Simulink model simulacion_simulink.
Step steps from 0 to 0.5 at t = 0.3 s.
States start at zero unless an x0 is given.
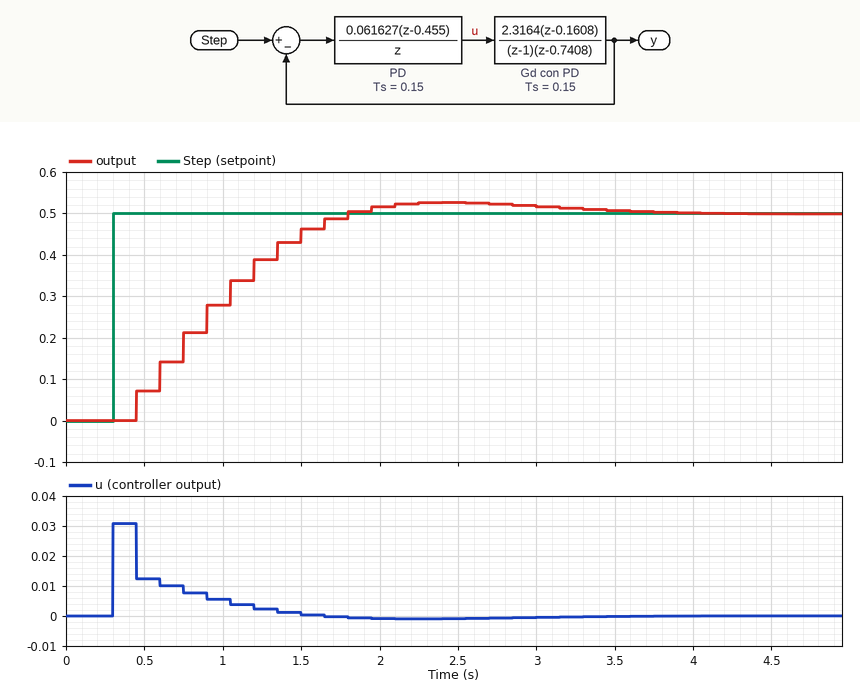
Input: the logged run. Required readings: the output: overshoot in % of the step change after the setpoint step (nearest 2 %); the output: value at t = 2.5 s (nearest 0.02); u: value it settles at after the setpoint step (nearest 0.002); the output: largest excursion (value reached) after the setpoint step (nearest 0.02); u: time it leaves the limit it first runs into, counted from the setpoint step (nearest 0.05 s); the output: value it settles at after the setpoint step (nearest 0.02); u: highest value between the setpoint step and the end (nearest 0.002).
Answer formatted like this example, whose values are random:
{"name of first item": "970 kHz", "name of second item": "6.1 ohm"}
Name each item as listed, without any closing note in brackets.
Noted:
{"the output: overshoot in % of the step change after the setpoint step": "6 %", "the output: value at t = 2.5 s": "0.52", "u: value it settles at after the setpoint step": "0.000", "the output: largest excursion (value reached) after the setpoint step": "0.52", "u: time it leaves the limit it first runs into, counted from the setpoint step": "0.15 s", "the output: value it settles at after the setpoint step": "0.50", "u: highest value between the setpoint step and the end": "0.030"}
